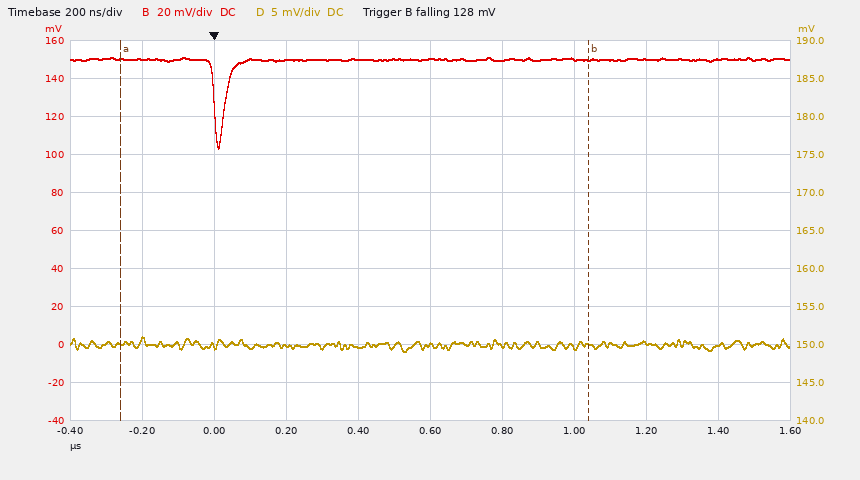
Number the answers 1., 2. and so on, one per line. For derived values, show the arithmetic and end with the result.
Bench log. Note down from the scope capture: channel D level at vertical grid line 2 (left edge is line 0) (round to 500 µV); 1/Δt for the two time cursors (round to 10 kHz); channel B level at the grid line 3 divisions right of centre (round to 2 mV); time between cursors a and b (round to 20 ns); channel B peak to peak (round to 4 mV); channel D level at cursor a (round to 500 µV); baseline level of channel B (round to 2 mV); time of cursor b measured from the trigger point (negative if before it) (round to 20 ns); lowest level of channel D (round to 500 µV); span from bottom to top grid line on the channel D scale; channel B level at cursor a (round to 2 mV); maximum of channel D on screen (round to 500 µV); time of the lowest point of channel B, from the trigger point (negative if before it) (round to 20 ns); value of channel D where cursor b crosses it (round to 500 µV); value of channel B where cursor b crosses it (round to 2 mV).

1. 150.0 mV
2. 1 / 1.30 µs ≈ 770 kHz
3. 150 mV
4. 1.30 µs
5. 48 mV
6. 150.0 mV
7. 150 mV
8. +1.04 µs
9. 149.0 mV
10. 50 mV
11. 150 mV
12. 151.0 mV
13. +20 ns
14. 150.0 mV
15. 150 mV
